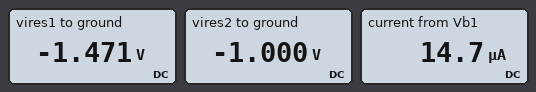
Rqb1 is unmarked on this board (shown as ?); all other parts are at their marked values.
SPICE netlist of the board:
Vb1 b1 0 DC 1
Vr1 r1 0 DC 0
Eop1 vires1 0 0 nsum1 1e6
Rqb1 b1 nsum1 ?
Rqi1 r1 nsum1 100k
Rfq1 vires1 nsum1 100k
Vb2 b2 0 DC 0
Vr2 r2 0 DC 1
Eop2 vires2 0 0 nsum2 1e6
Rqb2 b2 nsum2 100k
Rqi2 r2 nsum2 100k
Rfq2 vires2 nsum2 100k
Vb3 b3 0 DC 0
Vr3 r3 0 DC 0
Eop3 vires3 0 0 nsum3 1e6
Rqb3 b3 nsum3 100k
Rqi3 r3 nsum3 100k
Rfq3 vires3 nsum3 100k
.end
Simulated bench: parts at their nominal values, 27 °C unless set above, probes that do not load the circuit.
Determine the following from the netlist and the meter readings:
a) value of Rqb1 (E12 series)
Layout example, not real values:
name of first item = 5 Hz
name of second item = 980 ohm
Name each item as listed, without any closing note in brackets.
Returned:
value of Rqb1 = 68 kΩ
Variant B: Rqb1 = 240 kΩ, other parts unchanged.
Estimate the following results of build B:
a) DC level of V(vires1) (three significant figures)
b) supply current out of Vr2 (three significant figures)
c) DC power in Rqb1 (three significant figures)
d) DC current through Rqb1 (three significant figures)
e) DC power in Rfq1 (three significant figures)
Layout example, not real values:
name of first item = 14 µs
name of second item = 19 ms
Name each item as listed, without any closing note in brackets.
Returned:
DC level of V(vires1) = -417 mV
supply current out of Vr2 = 10.0 µA
DC power in Rqb1 = 4.17 µW
DC current through Rqb1 = 4.17 µA
DC power in Rfq1 = 1.74 µW
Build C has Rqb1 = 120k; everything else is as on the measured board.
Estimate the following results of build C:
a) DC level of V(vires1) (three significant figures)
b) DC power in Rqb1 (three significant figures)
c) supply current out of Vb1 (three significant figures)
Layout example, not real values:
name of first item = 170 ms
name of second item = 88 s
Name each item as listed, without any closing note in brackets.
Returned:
DC level of V(vires1) = -833 mV
DC power in Rqb1 = 8.33 µW
supply current out of Vb1 = 8.33 µA
